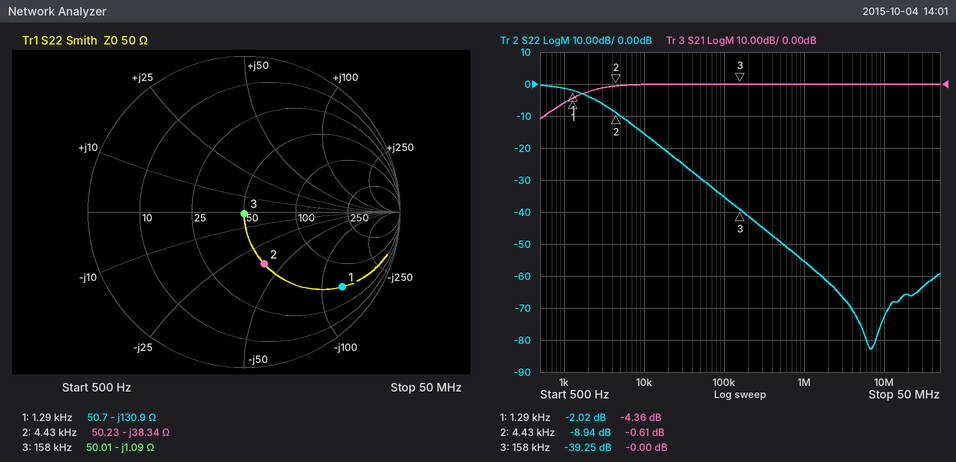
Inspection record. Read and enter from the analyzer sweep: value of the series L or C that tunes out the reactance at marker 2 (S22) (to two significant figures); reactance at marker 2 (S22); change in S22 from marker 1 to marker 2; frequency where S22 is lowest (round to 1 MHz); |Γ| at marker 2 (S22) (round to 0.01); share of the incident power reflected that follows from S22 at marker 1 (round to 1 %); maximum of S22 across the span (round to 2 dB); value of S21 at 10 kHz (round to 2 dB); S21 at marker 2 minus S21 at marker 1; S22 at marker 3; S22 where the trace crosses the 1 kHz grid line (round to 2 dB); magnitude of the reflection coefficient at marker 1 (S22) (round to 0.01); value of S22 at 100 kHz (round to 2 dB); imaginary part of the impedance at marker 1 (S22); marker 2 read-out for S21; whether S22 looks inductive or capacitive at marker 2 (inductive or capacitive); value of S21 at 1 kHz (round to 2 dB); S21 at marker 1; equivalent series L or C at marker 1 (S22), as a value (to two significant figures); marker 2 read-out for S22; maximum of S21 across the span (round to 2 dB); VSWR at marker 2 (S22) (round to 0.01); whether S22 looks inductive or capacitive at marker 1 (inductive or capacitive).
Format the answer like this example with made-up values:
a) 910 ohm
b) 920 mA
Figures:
a) 1.4 mH
b) -38.34 Ω
c) -6.92 dB
d) 7 MHz
e) 0.36
f) 63 %
g) 0 dB
h) 0 dB
i) 3.75 dB
j) -39.25 dB
k) -2 dB
l) 0.79
m) -36 dB
n) -130.9 Ω
o) -0.61 dB
p) capacitive
q) -6 dB
r) -4.36 dB
s) 940 nF
t) -8.94 dB
u) 0 dB
v) 2.11
w) capacitive
